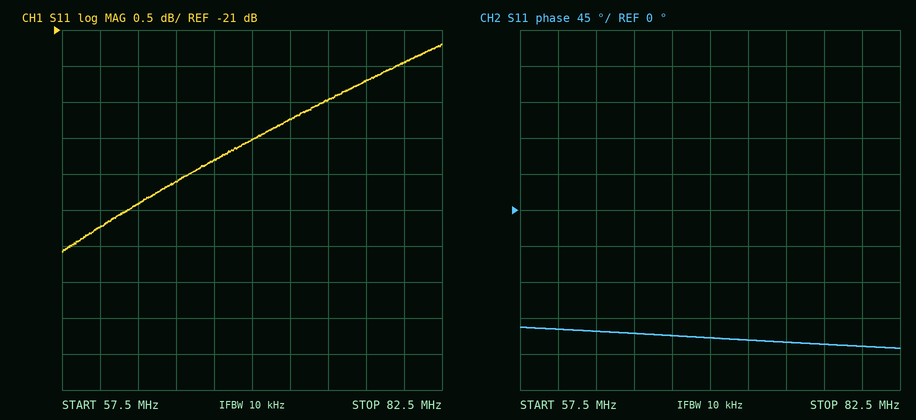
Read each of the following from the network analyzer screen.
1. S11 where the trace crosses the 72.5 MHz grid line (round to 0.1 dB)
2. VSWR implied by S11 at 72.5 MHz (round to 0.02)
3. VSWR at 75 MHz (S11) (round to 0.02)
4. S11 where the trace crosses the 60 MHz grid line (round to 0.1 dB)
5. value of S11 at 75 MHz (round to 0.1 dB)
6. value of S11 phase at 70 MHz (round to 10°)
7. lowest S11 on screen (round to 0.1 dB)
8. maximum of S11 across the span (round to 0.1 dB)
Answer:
-22.2 dB
1.16
1.18
-23.7 dB
-22.0 dB
-160°
-24.1 dB
-21.2 dB
